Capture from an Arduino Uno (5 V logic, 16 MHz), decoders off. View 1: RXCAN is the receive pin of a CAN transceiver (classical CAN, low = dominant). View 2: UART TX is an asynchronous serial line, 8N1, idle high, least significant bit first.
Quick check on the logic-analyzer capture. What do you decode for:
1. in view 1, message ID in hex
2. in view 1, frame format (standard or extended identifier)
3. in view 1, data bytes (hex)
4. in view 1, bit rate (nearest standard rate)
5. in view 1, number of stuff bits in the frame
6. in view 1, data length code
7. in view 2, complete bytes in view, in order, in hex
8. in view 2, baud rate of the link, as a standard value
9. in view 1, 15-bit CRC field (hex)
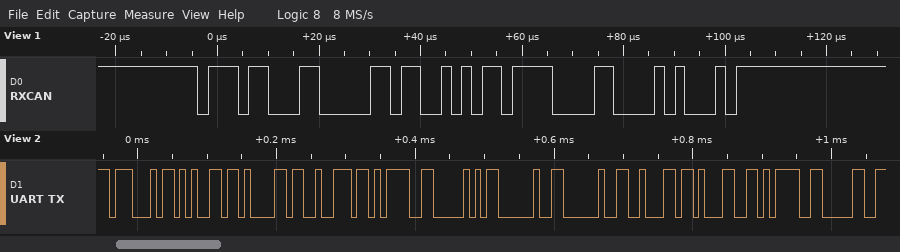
0x763
standard
CA DE
500 kbit/s
1
2
47 65 61 72 3D 50 20 20 62 31 3D 30
115200 baud
0x0C28
